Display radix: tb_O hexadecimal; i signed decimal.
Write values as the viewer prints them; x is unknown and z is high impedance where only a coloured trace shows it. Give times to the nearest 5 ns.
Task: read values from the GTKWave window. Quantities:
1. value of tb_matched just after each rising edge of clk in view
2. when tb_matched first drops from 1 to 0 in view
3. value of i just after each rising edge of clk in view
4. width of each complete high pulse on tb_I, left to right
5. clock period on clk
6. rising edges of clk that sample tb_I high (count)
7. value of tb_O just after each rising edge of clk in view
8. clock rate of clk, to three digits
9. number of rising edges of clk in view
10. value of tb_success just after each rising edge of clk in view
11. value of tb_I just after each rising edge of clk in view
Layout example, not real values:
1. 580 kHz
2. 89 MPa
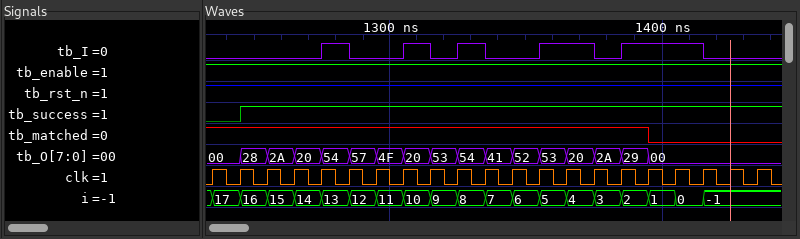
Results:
1. 1 1 1 1 1 1 1 1 1 1 1 1 1 1 1 1 0 0 0 0 0
2. 1395 ns
3. 17, 16, 15, 14, 13, 12, 11, 10, 9, 8, 7, 6, 5, 4, 3, 2, 1, 0, -1, -1, -1
4. 10 ns, 10 ns, 10 ns, 20 ns, 30 ns
5. 10 ns
6. 8
7. 00, 28, 2A, 20, 54, 57, 4F, 20, 53, 54, 41, 52, 53, 20, 2A, 29, 00, 00, 00, 00, 00
8. 100 MHz
9. 21
10. 0 1 1 1 1 1 1 1 1 1 1 1 1 1 1 1 1 1 1 1 1
11. 0 0 0 0 1 0 0 1 0 1 0 0 1 1 0 1 1 1 0 0 0
